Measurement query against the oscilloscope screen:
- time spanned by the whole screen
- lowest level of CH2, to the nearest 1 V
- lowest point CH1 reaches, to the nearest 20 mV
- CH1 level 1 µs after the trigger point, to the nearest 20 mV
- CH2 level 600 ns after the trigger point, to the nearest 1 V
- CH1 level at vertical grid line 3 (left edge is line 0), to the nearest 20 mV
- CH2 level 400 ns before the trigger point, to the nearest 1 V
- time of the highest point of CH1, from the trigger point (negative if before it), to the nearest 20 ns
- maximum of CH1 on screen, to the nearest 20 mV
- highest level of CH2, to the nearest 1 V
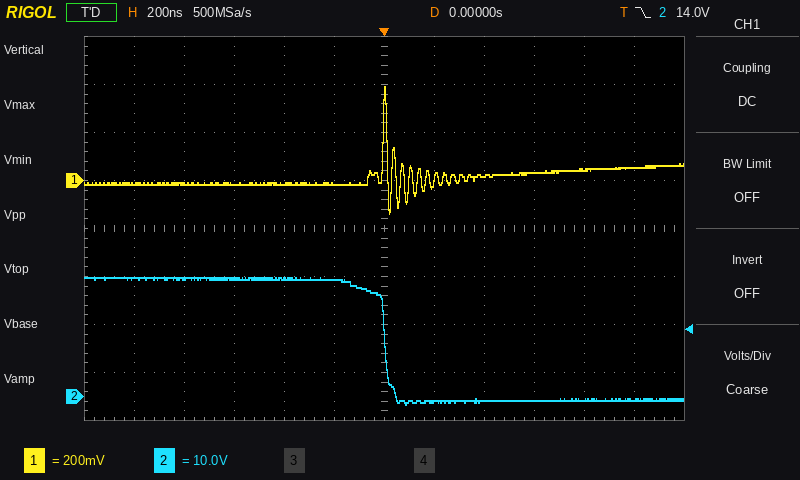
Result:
2.4 µs
-2 V
-140 mV
60 mV
-1 V
-20 mV
25 V
0 ns
400 mV
25 V
